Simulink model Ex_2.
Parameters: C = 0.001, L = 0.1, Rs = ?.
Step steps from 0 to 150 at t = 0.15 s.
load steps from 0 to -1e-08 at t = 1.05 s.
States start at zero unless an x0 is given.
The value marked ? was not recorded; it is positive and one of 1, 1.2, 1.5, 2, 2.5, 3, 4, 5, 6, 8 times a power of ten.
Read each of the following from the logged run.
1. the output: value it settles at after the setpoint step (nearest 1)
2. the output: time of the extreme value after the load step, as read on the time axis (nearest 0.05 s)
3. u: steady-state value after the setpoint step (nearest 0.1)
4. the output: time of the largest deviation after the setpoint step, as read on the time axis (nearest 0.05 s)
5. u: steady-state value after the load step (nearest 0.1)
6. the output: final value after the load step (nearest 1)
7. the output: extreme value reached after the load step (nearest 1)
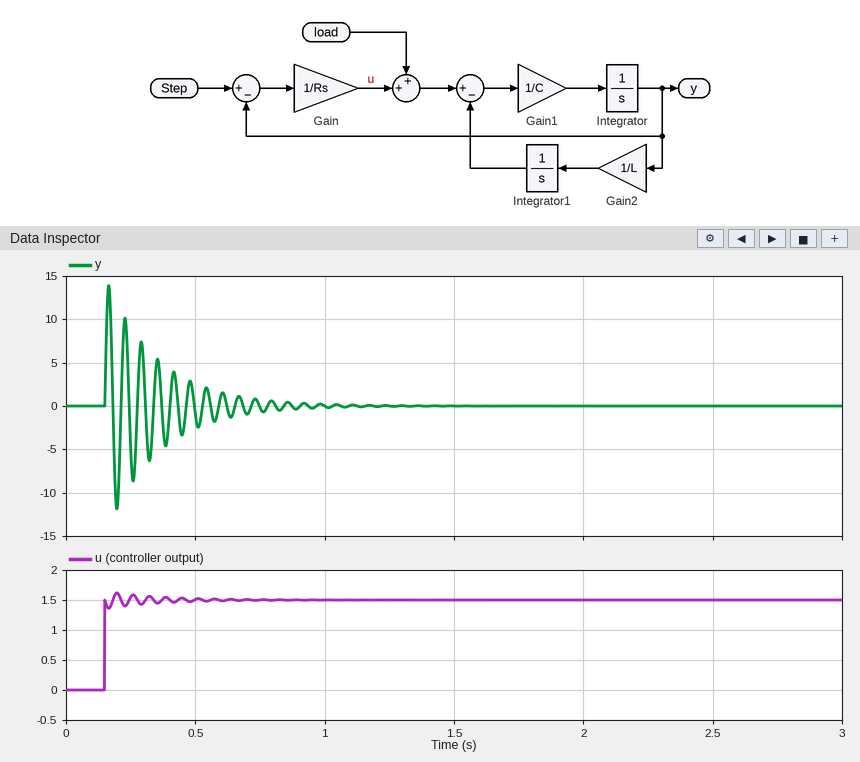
0
1.05 s
1.5
0.15 s
1.5
0
0
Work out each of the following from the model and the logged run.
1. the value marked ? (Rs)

100
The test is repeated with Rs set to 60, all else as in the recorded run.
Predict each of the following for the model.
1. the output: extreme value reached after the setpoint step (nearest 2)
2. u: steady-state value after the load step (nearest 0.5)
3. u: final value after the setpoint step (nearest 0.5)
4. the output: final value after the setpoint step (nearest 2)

22
2.5
2.5
0
